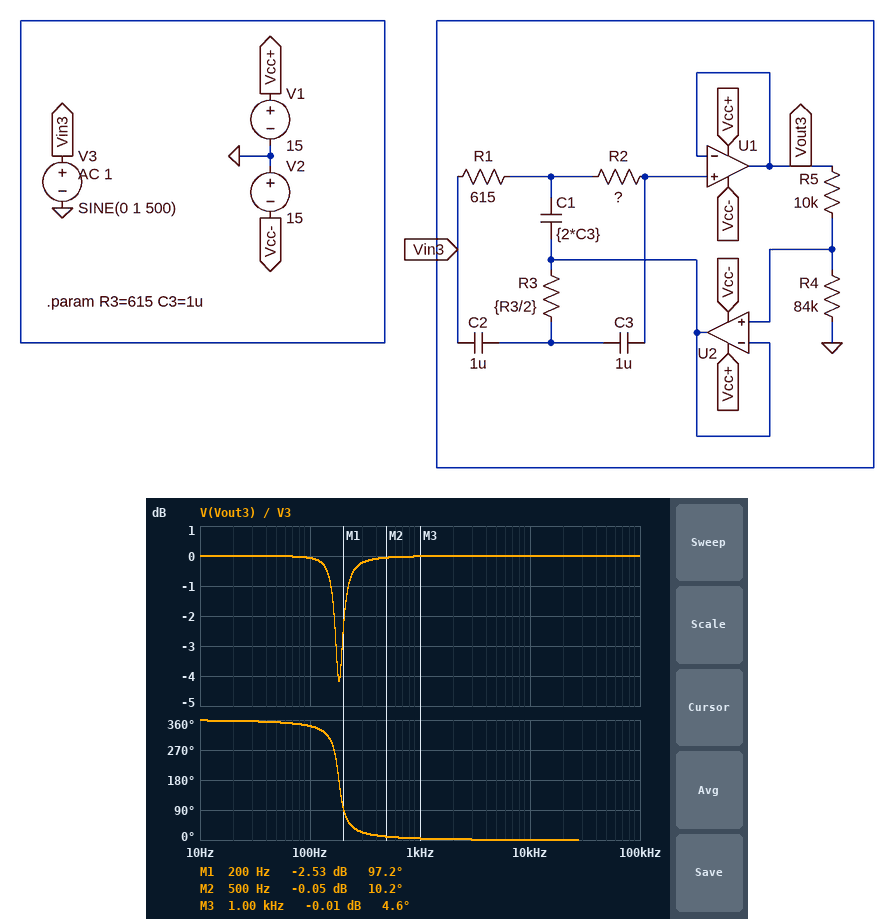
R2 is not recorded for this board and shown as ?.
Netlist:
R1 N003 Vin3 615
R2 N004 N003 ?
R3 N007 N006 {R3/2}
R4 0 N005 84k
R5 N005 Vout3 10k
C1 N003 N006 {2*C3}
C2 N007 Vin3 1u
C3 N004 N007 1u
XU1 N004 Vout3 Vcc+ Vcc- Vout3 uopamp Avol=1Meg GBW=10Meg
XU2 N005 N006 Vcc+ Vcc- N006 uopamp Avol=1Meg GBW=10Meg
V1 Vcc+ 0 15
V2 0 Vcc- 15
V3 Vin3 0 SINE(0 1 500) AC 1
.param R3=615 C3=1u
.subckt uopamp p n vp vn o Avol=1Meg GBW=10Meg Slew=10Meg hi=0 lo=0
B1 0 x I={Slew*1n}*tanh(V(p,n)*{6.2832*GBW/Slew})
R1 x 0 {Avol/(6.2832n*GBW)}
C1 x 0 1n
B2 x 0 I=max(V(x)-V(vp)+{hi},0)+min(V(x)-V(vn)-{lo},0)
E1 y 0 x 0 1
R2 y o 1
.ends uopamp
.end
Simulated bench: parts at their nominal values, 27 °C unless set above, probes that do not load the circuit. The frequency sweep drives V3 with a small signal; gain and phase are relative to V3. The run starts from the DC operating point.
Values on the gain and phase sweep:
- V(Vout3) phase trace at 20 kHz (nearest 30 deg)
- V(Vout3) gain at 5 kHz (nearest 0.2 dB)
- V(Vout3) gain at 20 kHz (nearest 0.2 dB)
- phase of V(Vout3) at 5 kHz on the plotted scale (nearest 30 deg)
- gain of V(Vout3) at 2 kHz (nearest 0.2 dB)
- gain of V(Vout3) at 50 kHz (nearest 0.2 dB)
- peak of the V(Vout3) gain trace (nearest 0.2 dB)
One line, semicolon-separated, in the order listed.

0 deg; 0 dB; 0 dB; 0 deg; 0 dB; 0 dB; 0 dB
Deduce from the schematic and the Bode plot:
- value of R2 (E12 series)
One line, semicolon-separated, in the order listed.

1.5 kΩ
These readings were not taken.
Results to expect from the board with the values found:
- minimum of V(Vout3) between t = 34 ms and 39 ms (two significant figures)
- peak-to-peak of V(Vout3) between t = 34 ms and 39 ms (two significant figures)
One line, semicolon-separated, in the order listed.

-990 mV; 2.0 V
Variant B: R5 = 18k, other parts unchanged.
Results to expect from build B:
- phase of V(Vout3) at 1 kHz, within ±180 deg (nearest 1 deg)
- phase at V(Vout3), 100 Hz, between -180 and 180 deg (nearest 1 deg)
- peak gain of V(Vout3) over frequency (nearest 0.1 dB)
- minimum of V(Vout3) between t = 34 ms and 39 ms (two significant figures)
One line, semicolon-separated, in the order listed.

8 deg; -29 deg; 0 dB; -970 mV
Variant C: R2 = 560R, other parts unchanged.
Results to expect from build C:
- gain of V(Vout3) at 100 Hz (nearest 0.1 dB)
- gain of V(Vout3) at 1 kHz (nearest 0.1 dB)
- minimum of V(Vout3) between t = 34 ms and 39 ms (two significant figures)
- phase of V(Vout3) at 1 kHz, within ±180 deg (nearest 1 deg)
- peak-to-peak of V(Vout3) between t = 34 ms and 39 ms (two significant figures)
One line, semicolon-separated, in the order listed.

-0.2 dB; -0.1 dB; -950 mV; 7 deg; 1.9 V
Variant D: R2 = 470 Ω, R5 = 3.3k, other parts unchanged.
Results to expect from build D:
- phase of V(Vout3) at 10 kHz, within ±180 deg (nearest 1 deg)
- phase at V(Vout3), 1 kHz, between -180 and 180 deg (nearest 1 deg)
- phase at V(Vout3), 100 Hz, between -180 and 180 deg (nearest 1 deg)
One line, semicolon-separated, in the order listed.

0 deg; 3 deg; -4 deg
